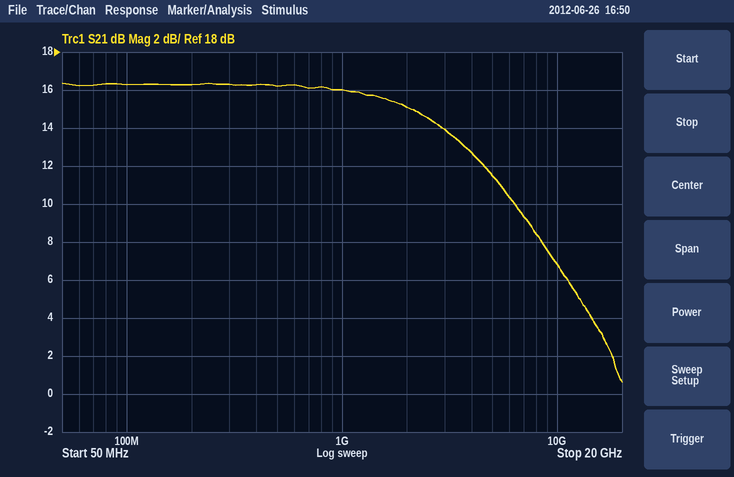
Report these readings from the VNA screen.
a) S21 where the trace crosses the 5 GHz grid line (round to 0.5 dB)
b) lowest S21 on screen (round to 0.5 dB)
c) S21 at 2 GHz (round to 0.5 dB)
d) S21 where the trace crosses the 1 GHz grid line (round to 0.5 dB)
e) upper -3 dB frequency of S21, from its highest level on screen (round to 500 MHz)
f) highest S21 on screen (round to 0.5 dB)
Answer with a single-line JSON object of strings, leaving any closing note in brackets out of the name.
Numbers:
{"S21 where the trace crosses the 5 GHz grid line": "11.5 dB", "lowest S21 on screen": "0.5 dB", "S21 at 2 GHz": "15.0 dB", "S21 where the trace crosses the 1 GHz grid line": "16.0 dB", "upper -3 dB frequency of S21, from its highest level on screen": "3.5 GHz", "highest S21 on screen": "16.5 dB"}
